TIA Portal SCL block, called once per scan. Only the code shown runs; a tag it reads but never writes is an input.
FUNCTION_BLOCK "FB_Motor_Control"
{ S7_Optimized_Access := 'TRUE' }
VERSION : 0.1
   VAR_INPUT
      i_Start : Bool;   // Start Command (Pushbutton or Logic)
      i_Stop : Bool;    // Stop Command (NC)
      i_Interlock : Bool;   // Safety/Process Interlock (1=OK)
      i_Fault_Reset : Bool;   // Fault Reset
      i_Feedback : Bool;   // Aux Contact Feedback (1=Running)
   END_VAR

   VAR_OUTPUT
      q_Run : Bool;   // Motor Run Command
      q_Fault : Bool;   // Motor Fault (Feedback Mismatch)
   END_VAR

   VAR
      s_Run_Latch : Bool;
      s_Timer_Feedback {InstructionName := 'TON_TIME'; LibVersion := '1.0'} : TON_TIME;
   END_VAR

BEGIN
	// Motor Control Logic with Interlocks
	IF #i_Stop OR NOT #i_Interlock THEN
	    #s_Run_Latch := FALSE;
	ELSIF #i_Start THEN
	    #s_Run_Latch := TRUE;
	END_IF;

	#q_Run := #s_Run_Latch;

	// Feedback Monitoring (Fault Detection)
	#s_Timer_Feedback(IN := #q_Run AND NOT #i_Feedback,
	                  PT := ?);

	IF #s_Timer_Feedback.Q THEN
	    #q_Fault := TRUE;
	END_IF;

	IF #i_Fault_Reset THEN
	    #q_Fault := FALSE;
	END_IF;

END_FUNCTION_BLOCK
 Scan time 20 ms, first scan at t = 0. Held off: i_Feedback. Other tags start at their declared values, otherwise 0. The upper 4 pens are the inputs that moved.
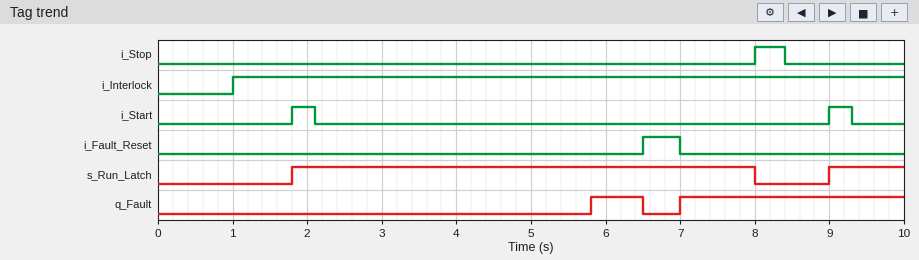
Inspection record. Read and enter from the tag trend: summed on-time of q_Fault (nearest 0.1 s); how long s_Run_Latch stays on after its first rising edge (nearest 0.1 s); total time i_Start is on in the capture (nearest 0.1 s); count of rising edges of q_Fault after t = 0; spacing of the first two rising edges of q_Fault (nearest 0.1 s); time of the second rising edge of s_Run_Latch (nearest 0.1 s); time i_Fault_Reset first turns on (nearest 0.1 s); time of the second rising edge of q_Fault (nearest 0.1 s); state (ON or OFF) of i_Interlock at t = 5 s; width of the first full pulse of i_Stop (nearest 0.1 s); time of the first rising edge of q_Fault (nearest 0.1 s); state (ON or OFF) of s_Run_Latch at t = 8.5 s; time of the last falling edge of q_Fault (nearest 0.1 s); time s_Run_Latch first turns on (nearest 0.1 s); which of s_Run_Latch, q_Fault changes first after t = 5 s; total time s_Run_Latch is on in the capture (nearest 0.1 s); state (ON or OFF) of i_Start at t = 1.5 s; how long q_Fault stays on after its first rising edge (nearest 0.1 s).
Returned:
3.7 s
6.2 s
0.6 s
2
1.2 s
9.0 s
6.5 s
7.0 s
ON
0.4 s
5.8 s
OFF
6.5 s
1.8 s
q_Fault
7.2 s
OFF
0.7 s
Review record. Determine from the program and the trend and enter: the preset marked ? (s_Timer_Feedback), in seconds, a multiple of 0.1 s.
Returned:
4.0 s
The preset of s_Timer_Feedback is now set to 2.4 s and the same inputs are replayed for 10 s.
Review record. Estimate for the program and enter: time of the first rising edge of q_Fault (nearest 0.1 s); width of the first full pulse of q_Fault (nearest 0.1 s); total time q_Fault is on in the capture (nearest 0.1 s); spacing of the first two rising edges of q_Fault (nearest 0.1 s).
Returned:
4.2 s
2.3 s
5.3 s
2.8 s
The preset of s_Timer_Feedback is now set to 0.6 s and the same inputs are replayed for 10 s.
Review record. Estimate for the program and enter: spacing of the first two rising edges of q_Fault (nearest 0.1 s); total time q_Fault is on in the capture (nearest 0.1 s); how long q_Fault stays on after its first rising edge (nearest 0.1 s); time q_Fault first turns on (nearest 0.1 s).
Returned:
4.6 s
7.1 s
4.1 s
2.4 s
